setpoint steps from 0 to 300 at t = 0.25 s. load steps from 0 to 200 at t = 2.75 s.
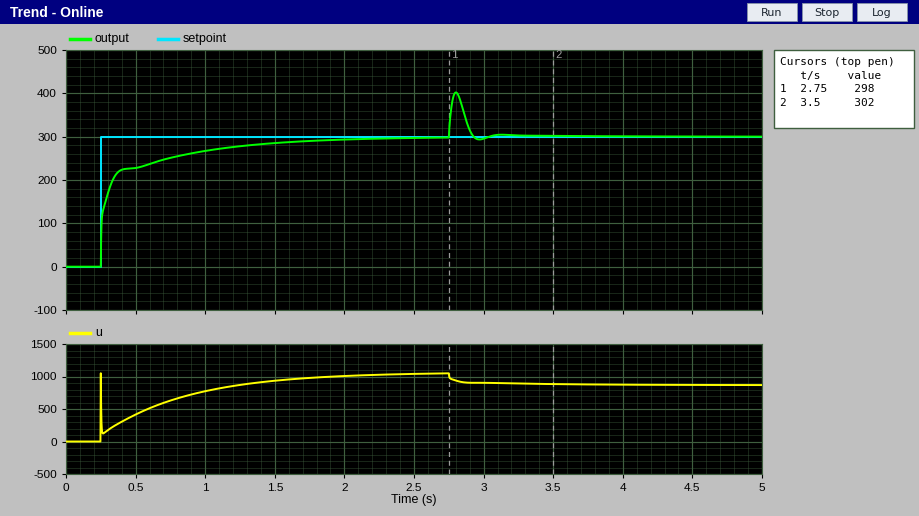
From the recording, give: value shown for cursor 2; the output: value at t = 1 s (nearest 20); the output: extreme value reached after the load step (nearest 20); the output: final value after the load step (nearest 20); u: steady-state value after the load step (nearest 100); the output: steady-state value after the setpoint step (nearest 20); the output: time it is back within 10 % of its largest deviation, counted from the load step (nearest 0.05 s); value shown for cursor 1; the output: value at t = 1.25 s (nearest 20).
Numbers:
302
260
400
300
900
300
0.15 s
298
280
